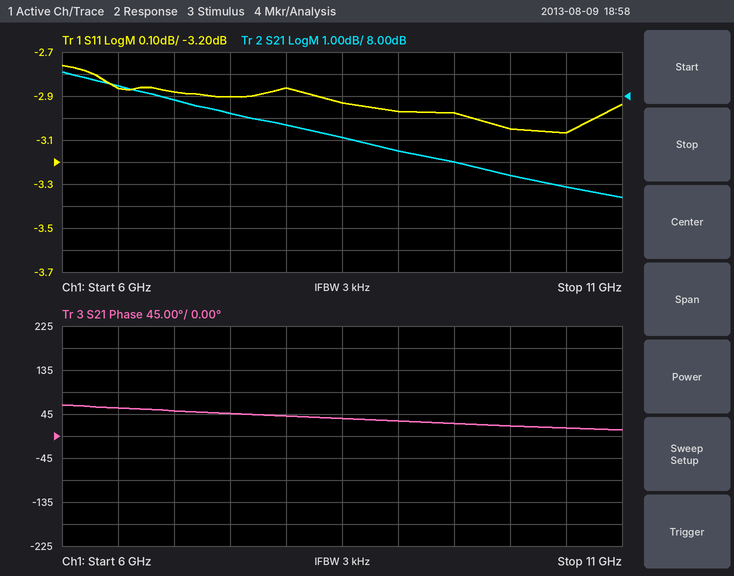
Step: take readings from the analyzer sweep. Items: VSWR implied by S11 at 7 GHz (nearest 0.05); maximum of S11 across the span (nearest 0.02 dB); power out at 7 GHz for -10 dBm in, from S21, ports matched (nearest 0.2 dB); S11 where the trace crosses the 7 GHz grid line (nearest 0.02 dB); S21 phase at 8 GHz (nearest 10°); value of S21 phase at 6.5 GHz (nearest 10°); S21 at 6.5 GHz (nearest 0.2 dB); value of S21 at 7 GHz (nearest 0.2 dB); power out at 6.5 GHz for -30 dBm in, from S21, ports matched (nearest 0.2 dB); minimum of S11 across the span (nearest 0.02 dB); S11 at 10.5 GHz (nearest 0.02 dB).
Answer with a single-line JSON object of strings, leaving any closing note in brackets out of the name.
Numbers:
{"VSWR implied by S11 at 7 GHz": "6.10", "maximum of S11 across the span": "-2.76 dB", "power out at 7 GHz for -10 dBm in, from S21, ports matched": "-2.2 dBm", "S11 where the trace crosses the 7 GHz grid line": "-2.88 dB", "S21 phase at 8 GHz": "40°", "value of S21 phase at 6.5 GHz": "60°", "S21 at 6.5 GHz": "8.4 dB", "value of S21 at 7 GHz": "7.8 dB", "power out at 6.5 GHz for -30 dBm in, from S21, ports matched": "-21.6 dBm", "minimum of S11 across the span": "-3.06 dB", "S11 at 10.5 GHz": "-3.06 dB"}
